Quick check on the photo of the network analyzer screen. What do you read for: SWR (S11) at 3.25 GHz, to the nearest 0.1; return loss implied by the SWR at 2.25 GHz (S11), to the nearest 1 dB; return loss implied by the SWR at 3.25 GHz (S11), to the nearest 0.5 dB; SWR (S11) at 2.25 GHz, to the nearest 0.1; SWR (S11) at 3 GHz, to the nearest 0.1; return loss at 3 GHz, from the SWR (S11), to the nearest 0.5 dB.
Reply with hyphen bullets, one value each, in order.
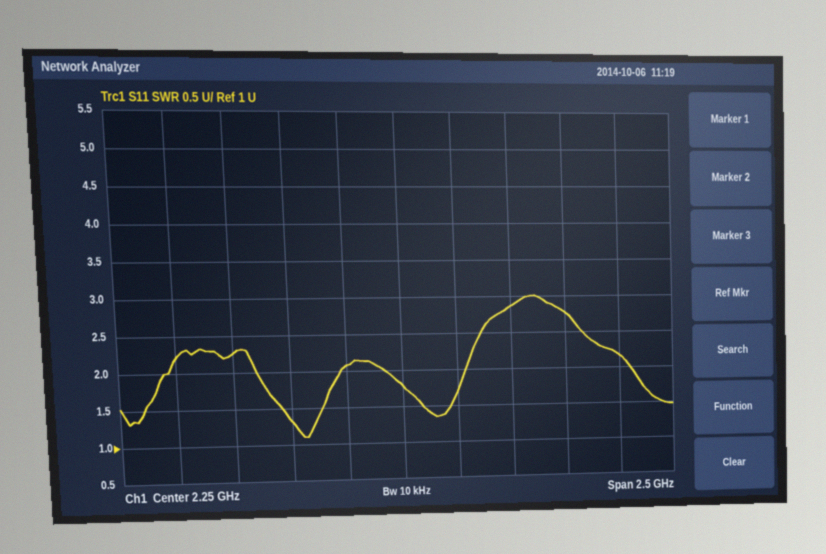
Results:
- 2.2
- 11 dB
- 8.5 dB
- 1.8
- 2.8
- 6.5 dB
